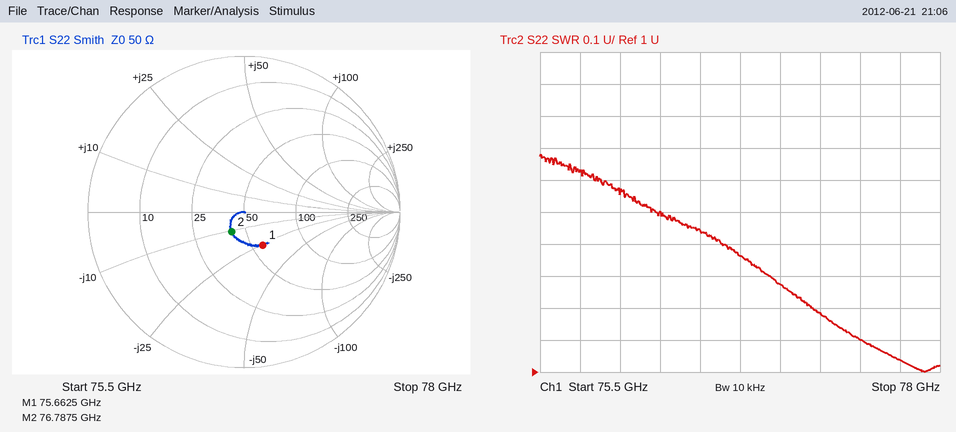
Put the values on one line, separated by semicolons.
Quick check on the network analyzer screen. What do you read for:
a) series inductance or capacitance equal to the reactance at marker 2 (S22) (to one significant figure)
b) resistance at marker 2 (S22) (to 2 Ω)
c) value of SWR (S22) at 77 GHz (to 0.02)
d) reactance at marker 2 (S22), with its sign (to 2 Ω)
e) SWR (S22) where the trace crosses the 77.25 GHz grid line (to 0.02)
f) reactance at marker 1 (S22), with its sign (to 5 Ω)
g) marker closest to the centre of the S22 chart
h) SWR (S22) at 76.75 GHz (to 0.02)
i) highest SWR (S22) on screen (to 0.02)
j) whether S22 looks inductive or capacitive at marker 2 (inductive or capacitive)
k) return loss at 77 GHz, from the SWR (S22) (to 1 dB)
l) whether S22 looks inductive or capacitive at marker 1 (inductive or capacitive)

200 fF; 42 Ω; 1.28; -10 Ω; 1.18; -25 Ω; marker 2; 1.36; 1.68; capacitive; 18 dB; capacitive
